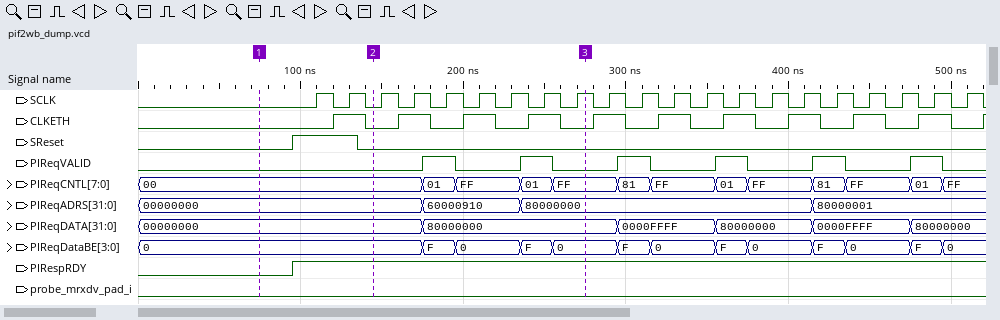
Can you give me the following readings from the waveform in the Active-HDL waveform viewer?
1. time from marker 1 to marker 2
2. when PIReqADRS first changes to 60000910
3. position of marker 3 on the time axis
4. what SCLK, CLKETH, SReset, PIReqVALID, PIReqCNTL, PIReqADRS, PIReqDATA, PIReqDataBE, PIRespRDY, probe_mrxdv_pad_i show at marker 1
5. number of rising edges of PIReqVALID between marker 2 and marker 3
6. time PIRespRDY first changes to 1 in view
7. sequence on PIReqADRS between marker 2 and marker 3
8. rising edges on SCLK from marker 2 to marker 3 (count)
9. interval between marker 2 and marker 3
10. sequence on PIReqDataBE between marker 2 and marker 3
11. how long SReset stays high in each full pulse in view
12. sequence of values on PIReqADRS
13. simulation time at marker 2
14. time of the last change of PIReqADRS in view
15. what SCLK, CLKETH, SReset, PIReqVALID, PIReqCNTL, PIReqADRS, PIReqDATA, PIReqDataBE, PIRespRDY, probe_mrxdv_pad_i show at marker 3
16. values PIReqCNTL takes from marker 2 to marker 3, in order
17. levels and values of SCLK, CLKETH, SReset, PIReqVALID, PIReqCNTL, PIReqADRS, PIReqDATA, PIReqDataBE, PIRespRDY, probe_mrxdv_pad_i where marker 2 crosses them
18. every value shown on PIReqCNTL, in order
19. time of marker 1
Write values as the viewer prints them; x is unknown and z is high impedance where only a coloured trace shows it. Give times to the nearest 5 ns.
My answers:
70 ns
175 ns
275 ns
SCLK=0, CLKETH=0, SReset=0, PIReqVALID=0, PIReqCNTL=00, PIReqADRS=00000000, PIReqDATA=00000000, PIReqDataBE=0, PIRespRDY=0, probe_mrxdv_pad_i=0
2
95 ns
00000000, 60000910, 80000000
7
130 ns
0, F, 0, F, 0
40 ns
00000000, 60000910, 80000000, 80000001
145 ns
415 ns
SCLK=1, CLKETH=0, SReset=0, PIReqVALID=0, PIReqCNTL=FF, PIReqADRS=80000000, PIReqDATA=80000000, PIReqDataBE=0, PIRespRDY=1, probe_mrxdv_pad_i=0
00, 01, FF, 01, FF
SCLK=0, CLKETH=0, SReset=0, PIReqVALID=0, PIReqCNTL=00, PIReqADRS=00000000, PIReqDATA=00000000, PIReqDataBE=0, PIRespRDY=1, probe_mrxdv_pad_i=0
00, 01, FF, 01, FF, 81, FF, 01, FF, 81, FF, 01, FF
75 ns
